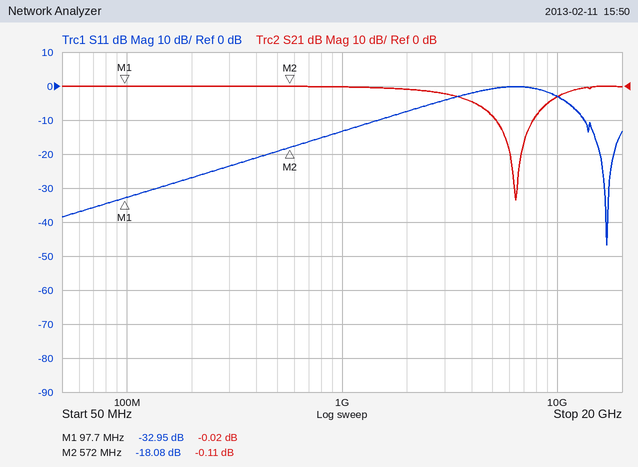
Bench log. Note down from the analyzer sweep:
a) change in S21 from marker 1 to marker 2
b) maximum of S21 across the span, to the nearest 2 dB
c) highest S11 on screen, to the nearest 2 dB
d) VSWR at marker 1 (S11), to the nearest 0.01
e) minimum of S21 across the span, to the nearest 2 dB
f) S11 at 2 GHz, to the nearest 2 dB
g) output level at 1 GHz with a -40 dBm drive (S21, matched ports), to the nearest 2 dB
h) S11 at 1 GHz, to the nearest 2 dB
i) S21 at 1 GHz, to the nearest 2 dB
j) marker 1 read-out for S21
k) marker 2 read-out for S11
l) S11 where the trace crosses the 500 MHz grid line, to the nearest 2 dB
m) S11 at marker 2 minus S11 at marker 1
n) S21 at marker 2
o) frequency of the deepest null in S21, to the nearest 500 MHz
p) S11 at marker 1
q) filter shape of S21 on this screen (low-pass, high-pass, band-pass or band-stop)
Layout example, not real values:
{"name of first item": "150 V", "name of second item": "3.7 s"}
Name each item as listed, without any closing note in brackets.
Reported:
{"change in S21 from marker 1 to marker 2": "-0.09 dB", "maximum of S21 across the span, to the nearest 2 dB": "0 dB", "highest S11 on screen, to the nearest 2 dB": "0 dB", "VSWR at marker 1 (S11), to the nearest 0.01": "1.05", "minimum of S21 across the span, to the nearest 2 dB": "-34 dB", "S11 at 2 GHz, to the nearest 2 dB": "-8 dB", "output level at 1 GHz with a -40 dBm drive (S21, matched ports), to the nearest 2 dB": "-40 dBm", "S11 at 1 GHz, to the nearest 2 dB": "-14 dB", "S21 at 1 GHz, to the nearest 2 dB": "0 dB", "marker 1 read-out for S21": "-0.02 dB", "marker 2 read-out for S11": "-18.08 dB", "S11 where the trace crosses the 500 MHz grid line, to the nearest 2 dB": "-20 dB", "S11 at marker 2 minus S11 at marker 1": "14.87 dB", "S21 at marker 2": "-0.11 dB", "frequency of the deepest null in S21, to the nearest 500 MHz": "6.5 GHz", "S11 at marker 1": "-32.95 dB", "filter shape of S21 on this screen": "band-stop"}
